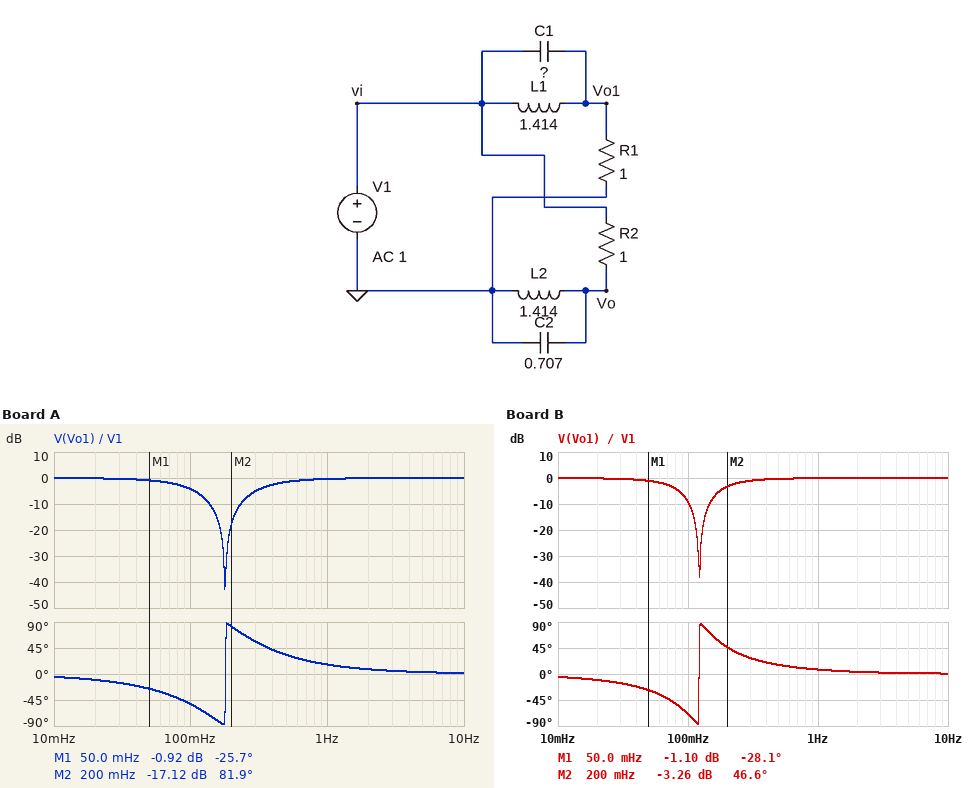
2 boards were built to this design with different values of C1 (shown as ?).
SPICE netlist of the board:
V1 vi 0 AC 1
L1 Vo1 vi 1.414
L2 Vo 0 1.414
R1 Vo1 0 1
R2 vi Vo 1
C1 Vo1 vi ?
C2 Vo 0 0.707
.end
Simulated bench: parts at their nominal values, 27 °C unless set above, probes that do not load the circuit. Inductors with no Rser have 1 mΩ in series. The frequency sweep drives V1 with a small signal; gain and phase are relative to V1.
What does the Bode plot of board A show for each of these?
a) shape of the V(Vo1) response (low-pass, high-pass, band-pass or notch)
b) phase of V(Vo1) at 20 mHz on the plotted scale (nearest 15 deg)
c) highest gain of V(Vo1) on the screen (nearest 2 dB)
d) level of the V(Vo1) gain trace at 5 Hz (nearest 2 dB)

notch
-15 deg
0 dB
0 dB
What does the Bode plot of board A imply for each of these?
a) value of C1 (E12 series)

560 mF
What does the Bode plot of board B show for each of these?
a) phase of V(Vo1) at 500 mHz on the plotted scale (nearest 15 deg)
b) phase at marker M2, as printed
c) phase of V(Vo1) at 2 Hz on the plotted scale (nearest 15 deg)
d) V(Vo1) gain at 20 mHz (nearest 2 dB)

15 deg
46.6 deg
0 deg
0 dB
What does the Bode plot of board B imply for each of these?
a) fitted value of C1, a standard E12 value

1.2 F
